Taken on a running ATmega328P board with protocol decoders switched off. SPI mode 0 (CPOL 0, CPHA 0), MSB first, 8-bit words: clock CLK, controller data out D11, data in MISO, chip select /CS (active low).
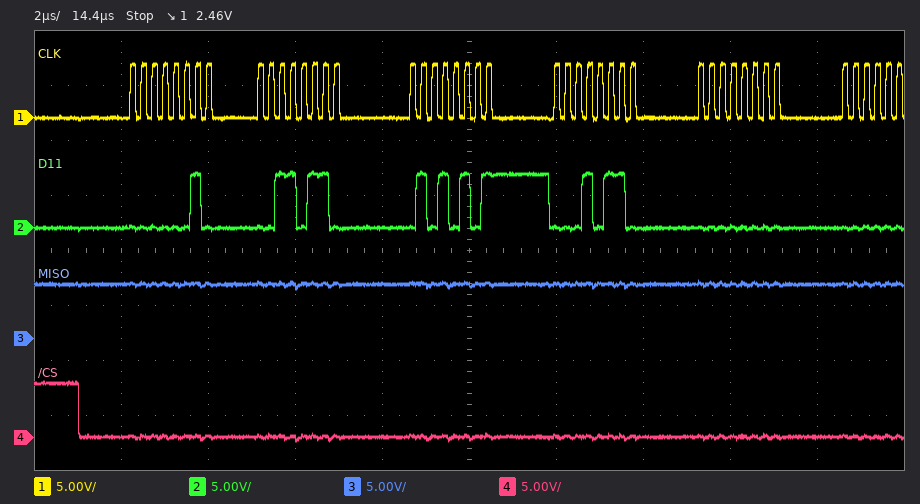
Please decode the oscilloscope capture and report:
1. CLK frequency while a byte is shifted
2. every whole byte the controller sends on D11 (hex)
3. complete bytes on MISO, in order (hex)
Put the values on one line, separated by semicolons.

4 MHz; 02 36 55 16 00; FF FF FF FF FF
